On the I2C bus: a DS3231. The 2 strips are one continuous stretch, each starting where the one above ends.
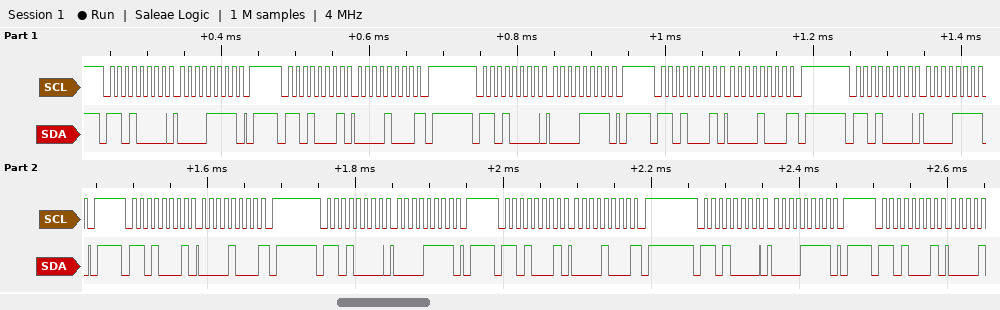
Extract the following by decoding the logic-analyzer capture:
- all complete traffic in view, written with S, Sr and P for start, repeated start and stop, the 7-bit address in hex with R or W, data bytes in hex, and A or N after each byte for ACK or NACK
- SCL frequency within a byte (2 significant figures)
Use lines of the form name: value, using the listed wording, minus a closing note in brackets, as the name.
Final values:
all complete traffic in view, written with S, Sr and P for start, repeated start and stop, the 7-bit address in hex with R or W, data bytes in hex, and A or N after each byte for ACK or NACK: S 68W A 0F A P S 68R A 08 N P S 68W A 0F A P S 68R A 08 N P S 68W A 0F A P S 68R A 08 N P S 68W A 0F A P S 68R A 08 N P S 68W A 0F A P S 68R A
SCL frequency within a byte: 100 kHz
